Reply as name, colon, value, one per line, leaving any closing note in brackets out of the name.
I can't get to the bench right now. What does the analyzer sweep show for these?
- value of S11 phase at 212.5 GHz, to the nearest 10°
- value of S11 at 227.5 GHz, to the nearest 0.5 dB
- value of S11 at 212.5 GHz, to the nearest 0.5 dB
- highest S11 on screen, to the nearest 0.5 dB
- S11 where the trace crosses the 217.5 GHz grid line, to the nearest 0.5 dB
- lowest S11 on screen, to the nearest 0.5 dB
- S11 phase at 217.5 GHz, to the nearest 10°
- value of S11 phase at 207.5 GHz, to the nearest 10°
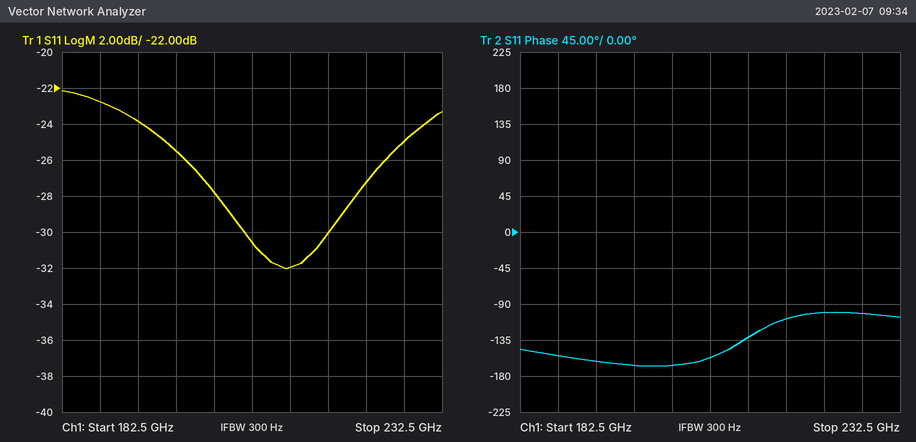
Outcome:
value of S11 phase at 212.5 GHz, to the nearest 10°: -130°
value of S11 at 227.5 GHz, to the nearest 0.5 dB: -25.0 dB
value of S11 at 212.5 GHz, to the nearest 0.5 dB: -32.0 dB
highest S11 on screen, to the nearest 0.5 dB: -22.0 dB
S11 where the trace crosses the 217.5 GHz grid line, to the nearest 0.5 dB: -30.0 dB
lowest S11 on screen, to the nearest 0.5 dB: -32.0 dB
S11 phase at 217.5 GHz, to the nearest 10°: -110°
value of S11 phase at 207.5 GHz, to the nearest 10°: -160°
